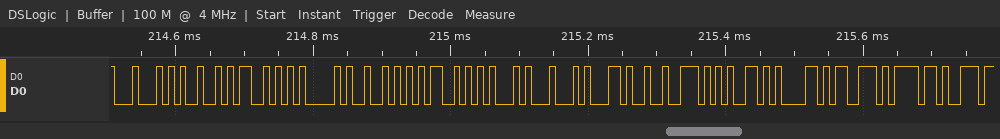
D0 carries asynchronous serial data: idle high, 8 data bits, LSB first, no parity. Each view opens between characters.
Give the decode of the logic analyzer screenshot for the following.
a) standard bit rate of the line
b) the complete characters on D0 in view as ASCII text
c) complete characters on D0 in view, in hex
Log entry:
115200 baud
"DISARMED,reaso"
44, 49, 53, 41, 52, 4D, 45, 44, 2C, 72, 65, 61, 73, 6F
